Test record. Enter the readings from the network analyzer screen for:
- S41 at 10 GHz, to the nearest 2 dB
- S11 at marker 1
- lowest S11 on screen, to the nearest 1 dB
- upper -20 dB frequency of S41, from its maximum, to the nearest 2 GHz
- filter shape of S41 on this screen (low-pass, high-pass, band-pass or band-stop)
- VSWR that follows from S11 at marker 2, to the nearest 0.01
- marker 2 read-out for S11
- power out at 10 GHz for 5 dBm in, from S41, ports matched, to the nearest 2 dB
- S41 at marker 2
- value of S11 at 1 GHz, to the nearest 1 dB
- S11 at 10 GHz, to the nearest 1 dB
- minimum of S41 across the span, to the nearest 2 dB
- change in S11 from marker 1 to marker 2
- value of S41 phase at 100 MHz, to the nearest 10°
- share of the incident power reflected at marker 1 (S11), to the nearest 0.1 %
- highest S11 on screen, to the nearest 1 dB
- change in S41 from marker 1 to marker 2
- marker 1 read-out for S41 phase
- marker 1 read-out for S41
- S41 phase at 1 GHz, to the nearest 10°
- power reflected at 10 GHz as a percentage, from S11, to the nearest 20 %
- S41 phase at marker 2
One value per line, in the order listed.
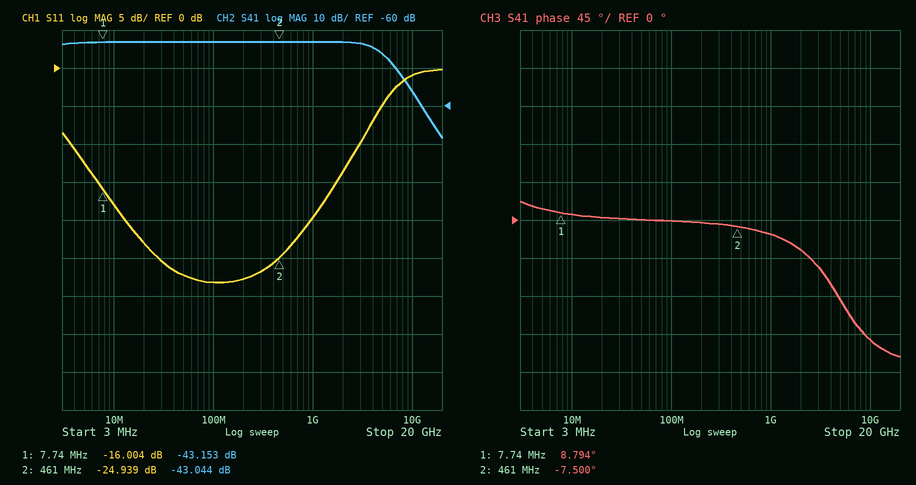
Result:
-56 dB
-16.004 dB
-28 dB
14 GHz
low-pass
1.12
-24.939 dB
-52 dBm
-43.044 dB
-20 dB
-1 dB
-68 dB
-8.935 dB
0°
2.5 %
0 dB
0.109 dB
8.794°
-43.153 dB
-20°
80 %
-7.500°
